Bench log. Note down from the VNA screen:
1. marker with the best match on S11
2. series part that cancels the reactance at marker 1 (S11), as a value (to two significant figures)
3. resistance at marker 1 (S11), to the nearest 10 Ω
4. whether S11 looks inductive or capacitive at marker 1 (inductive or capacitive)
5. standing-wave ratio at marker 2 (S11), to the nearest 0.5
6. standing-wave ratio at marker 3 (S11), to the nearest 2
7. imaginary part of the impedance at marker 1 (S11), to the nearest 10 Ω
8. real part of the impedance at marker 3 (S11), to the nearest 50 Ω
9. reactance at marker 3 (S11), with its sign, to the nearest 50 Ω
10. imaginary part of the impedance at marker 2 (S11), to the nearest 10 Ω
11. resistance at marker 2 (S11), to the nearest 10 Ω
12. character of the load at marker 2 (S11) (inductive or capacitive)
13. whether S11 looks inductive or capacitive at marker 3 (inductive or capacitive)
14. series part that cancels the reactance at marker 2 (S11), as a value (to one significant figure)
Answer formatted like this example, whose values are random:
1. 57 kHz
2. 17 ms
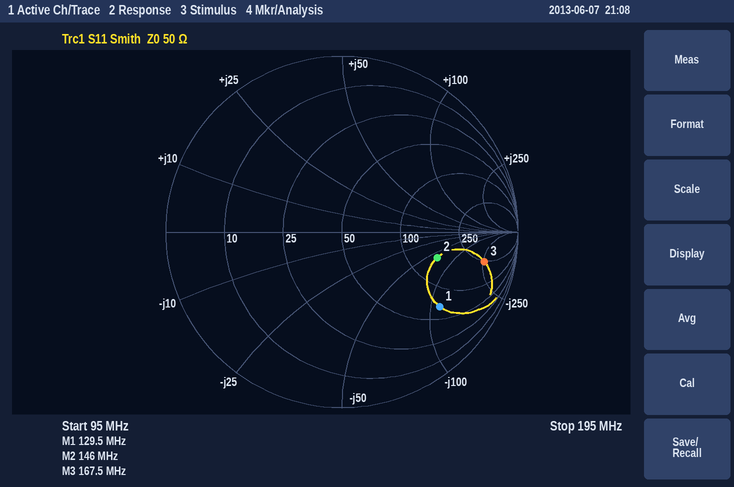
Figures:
1. marker 2
2. 140 nH
3. 70 Ω
4. capacitive
5. 3.5
6. 10
7. -110 Ω
8. 250 Ω
9. -250 Ω
10. -60 Ω
11. 150 Ω
12. capacitive
13. capacitive
14. 70 nH
